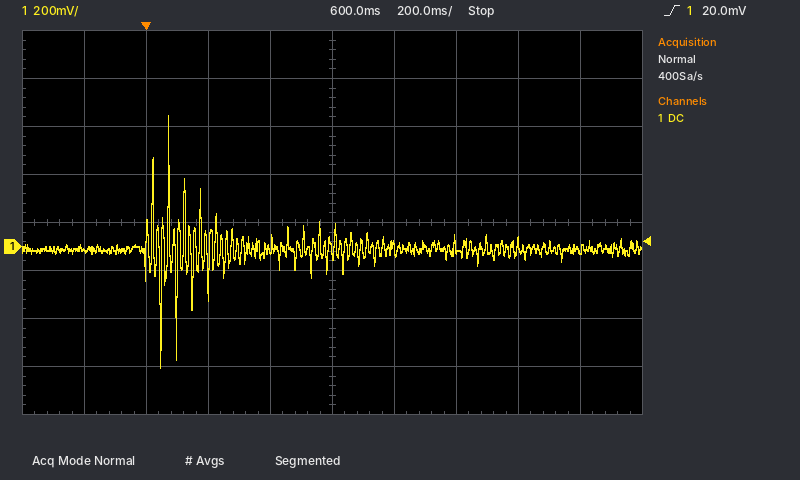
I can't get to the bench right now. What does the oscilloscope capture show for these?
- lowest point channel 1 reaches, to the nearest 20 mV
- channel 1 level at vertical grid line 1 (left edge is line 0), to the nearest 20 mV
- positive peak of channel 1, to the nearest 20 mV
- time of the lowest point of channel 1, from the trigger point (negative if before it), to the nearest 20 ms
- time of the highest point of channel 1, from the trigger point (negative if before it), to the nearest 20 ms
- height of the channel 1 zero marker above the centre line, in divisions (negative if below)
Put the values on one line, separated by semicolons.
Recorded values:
-500 mV; -20 mV; 540 mV; +40 ms; +80 ms; -0.5 div
